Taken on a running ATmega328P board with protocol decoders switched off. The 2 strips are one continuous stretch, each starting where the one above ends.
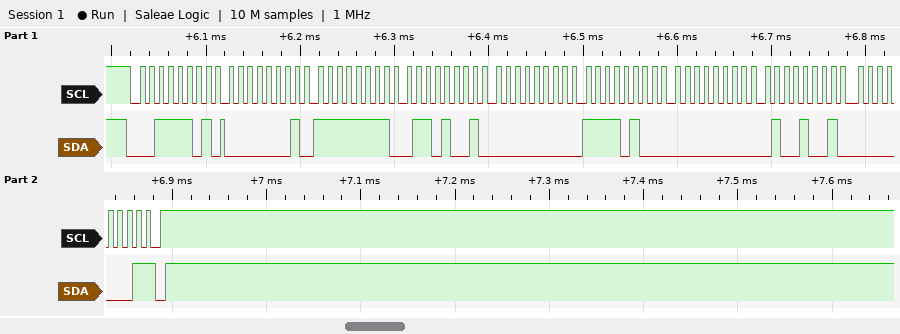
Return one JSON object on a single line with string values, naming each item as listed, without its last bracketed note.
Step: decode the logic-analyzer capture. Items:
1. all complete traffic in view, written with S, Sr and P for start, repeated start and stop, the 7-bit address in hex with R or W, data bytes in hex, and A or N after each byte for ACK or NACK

{"all complete traffic in view, written with S, Sr and P for start, repeated start and stop, the 7-bit address in hex with R or W, data bytes in hex, and A or N after each byte for ACK or NACK": "S 1ER A 01 A FF A 69 A 00 A F4 A 00 A 49 A 01 N P"}
